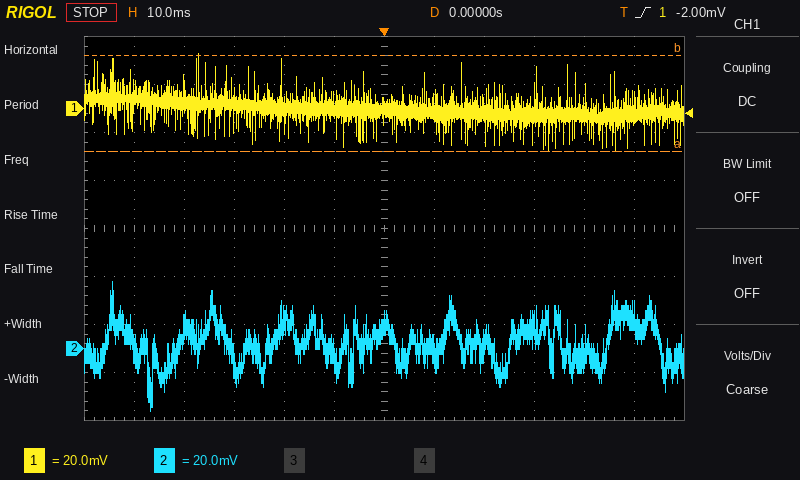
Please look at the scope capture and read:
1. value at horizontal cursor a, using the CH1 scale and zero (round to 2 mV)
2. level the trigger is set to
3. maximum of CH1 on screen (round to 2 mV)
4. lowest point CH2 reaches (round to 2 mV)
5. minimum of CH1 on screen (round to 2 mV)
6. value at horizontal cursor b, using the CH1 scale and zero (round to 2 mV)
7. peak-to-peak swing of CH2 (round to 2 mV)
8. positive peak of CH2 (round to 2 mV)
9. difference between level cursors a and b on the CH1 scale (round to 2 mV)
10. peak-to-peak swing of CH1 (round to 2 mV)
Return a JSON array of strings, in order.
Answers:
["-18 mV", "-2.00 mV", "22 mV", "-26 mV", "-18 mV", "22 mV", "54 mV", "28 mV", "40 mV", "40 mV"]
